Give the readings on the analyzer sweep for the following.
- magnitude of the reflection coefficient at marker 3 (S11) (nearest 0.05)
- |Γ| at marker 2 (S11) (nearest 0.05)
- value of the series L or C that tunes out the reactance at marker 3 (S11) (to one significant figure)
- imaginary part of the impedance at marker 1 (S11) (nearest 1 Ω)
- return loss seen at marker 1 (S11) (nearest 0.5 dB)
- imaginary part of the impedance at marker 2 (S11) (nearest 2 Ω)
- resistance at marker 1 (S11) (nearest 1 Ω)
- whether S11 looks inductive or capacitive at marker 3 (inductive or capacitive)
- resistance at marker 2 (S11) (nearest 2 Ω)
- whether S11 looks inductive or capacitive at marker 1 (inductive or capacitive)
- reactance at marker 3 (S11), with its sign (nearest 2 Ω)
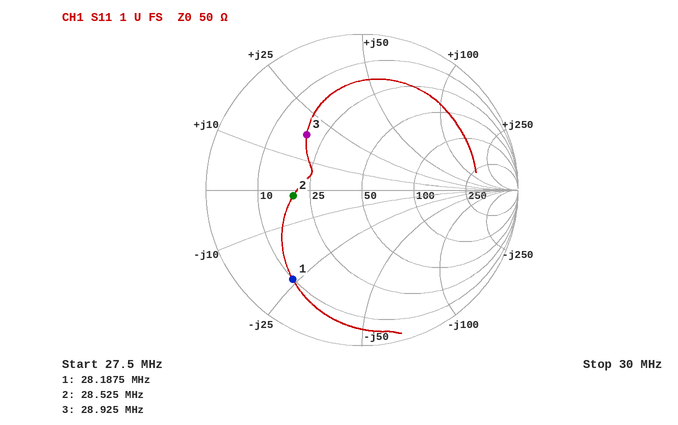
0.50
0.45
300 pF
-24 Ω
3.0 dB
-2 Ω
10 Ω
inductive
20 Ω
capacitive
+18 Ω
